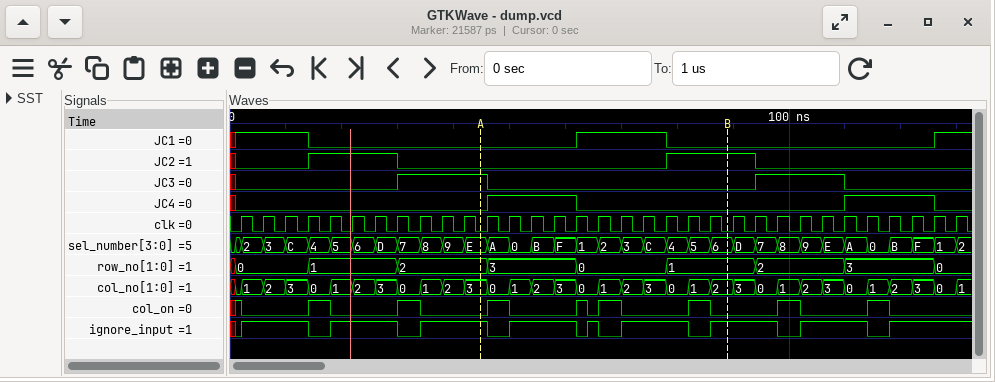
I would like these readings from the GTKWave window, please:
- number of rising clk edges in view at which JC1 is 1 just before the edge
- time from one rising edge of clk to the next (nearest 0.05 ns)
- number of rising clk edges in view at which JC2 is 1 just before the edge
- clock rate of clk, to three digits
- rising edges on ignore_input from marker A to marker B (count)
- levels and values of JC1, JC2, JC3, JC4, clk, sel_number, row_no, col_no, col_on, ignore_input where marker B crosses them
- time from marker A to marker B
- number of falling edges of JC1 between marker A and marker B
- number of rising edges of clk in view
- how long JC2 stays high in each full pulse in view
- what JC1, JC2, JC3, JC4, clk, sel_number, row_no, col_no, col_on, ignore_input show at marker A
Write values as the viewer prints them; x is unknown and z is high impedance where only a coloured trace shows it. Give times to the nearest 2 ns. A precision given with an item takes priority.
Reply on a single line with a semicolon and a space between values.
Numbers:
9; 4 ns; 8; 250 MHz; 4; JC1=0, JC2=1, JC3=0, JC4=0, clk=0, sel_number=6, row_no=1, col_no=2, col_on=0, ignore_input=1; 44 ns; 1; 33; 16 ns, 16 ns; JC1=0, JC2=0, JC3=1, JC4=0, clk=0, sel_number=E, row_no=2, col_no=3, col_on=0, ignore_input=1
